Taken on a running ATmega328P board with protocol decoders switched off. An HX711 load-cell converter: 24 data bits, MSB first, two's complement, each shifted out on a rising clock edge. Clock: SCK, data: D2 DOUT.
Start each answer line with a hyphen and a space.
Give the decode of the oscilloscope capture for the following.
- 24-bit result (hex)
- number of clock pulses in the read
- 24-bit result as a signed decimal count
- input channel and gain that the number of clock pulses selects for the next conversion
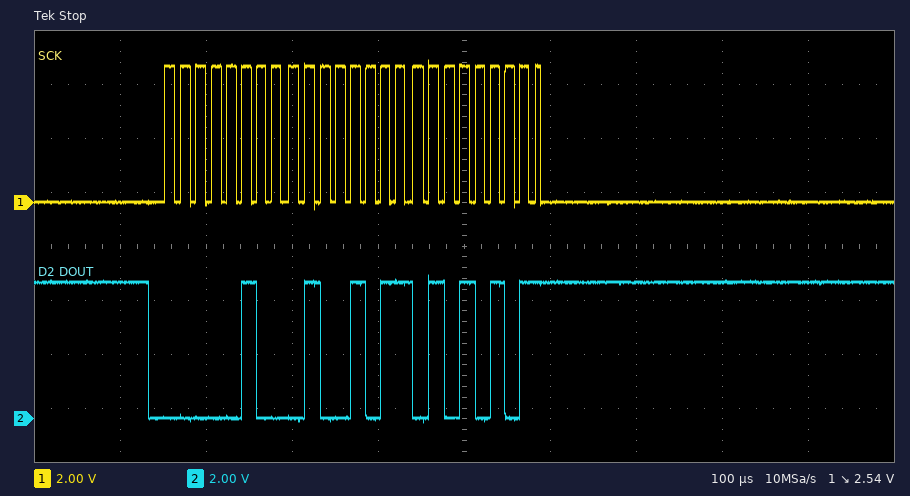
- 0x044B55
- 25
- 281429
- channel A, gain 128
